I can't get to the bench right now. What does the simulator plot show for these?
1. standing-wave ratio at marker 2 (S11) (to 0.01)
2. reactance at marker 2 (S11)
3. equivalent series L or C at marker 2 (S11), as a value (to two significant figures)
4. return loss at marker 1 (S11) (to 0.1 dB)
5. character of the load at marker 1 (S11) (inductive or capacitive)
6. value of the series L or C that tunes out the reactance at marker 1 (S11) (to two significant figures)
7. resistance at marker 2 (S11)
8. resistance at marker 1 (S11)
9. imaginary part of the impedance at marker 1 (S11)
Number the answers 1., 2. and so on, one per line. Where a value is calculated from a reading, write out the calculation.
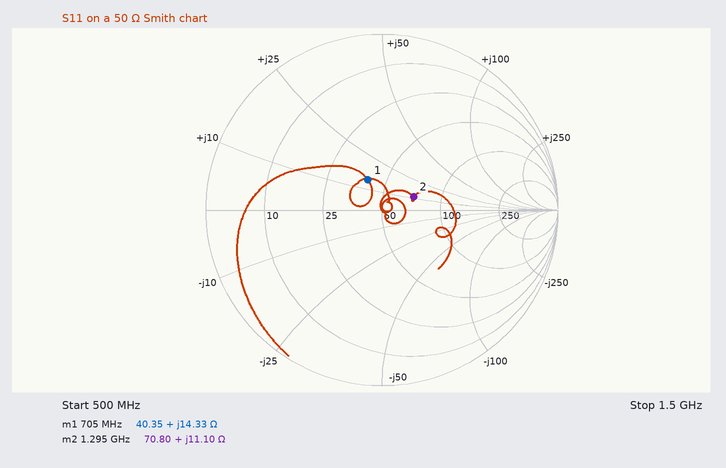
1. 1.48
2. +11.10 Ω
3. L = 11.1 Ω/(2π × 1.295 GHz) ≈ 1.4 nH
4. 14.5 dB
5. inductive
6. C = 1/(2π × 705 MHz × 14.33 Ω) ≈ 16 pF
7. 70.80 Ω
8. 40.35 Ω
9. +14.33 Ω
